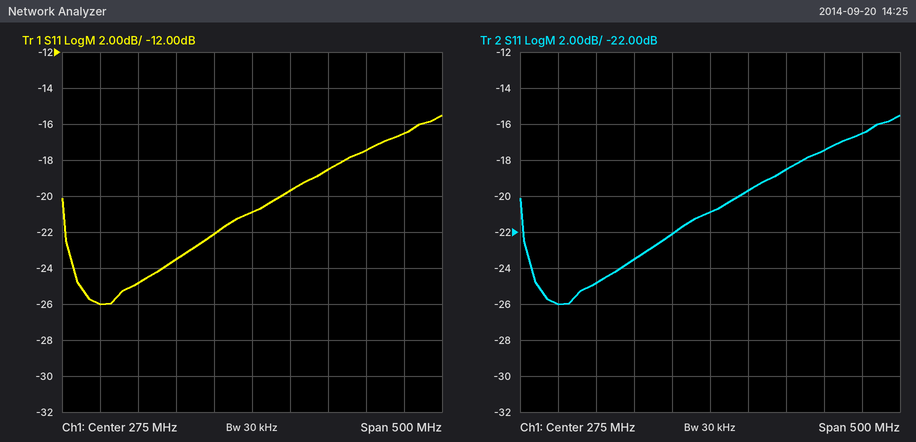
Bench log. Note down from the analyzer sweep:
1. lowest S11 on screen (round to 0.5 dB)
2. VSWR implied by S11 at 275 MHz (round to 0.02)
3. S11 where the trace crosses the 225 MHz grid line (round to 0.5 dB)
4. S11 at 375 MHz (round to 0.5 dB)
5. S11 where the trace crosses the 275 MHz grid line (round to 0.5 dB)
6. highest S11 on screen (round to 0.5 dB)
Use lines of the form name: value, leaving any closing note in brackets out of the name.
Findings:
lowest S11 on screen: -26.0 dB
VSWR implied by S11 at 275 MHz: 1.20
S11 where the trace crosses the 225 MHz grid line: -22.0 dB
S11 at 375 MHz: -18.5 dB
S11 where the trace crosses the 275 MHz grid line: -21.0 dB
highest S11 on screen: -15.5 dB
